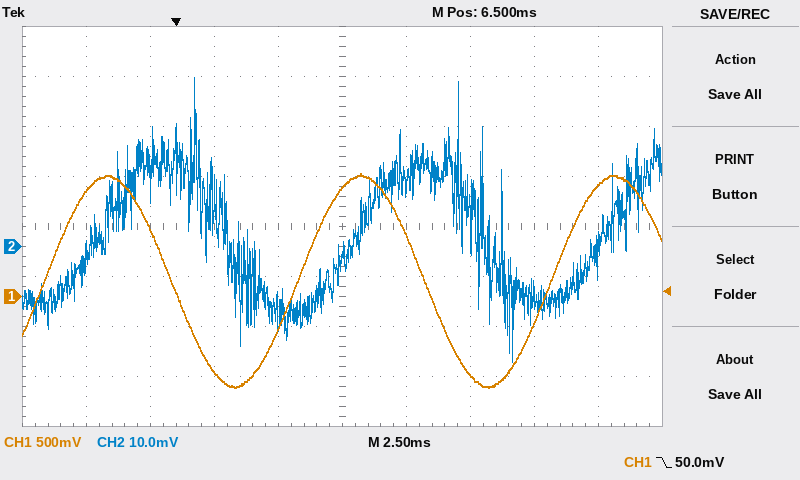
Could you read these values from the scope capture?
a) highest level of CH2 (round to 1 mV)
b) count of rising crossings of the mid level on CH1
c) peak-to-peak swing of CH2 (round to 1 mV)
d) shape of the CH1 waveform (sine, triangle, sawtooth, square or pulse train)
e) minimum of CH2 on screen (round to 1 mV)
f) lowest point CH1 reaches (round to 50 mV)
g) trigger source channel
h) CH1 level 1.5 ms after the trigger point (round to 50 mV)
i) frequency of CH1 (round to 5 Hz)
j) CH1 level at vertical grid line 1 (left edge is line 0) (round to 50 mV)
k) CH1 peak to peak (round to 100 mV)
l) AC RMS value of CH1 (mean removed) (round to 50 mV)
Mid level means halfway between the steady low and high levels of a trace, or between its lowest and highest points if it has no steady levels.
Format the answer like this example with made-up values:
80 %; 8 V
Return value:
34 mV; 3; 57 mV; sine; -23 mV; -900 mV; CH1; -750 mV; 100 Hz; 1.05 V; 2.10 V; 750 mV
